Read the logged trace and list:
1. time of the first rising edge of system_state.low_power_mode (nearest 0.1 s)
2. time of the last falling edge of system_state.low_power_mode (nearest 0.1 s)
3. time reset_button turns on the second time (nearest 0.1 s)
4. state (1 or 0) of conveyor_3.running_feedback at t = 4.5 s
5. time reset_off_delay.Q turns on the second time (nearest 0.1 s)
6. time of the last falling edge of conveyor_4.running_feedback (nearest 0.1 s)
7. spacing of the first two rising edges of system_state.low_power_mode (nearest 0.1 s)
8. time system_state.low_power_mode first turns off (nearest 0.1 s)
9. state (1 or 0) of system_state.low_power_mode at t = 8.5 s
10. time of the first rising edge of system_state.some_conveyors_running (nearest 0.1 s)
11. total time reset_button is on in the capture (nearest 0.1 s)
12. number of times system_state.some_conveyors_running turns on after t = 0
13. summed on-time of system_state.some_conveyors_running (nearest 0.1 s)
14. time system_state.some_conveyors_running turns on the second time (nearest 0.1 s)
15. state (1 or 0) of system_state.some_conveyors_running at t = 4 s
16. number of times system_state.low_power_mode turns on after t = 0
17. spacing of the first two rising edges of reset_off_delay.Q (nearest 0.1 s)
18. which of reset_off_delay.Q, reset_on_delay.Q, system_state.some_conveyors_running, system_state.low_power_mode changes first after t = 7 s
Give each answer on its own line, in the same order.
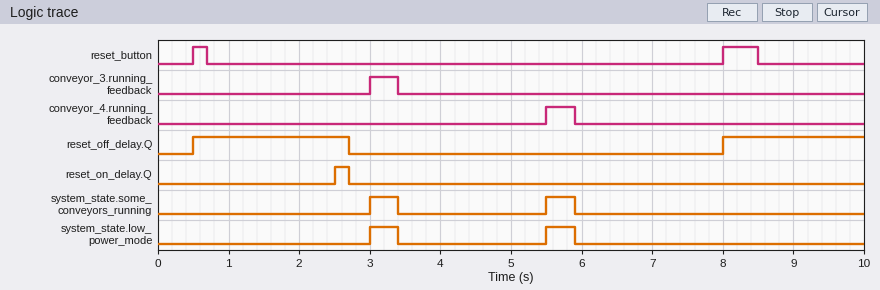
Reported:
3.0 s
5.9 s
8.0 s
0
8.0 s
5.9 s
2.5 s
3.4 s
0
3.0 s
0.7 s
2
0.8 s
5.5 s
0
2
7.5 s
reset_off_delay.Q
